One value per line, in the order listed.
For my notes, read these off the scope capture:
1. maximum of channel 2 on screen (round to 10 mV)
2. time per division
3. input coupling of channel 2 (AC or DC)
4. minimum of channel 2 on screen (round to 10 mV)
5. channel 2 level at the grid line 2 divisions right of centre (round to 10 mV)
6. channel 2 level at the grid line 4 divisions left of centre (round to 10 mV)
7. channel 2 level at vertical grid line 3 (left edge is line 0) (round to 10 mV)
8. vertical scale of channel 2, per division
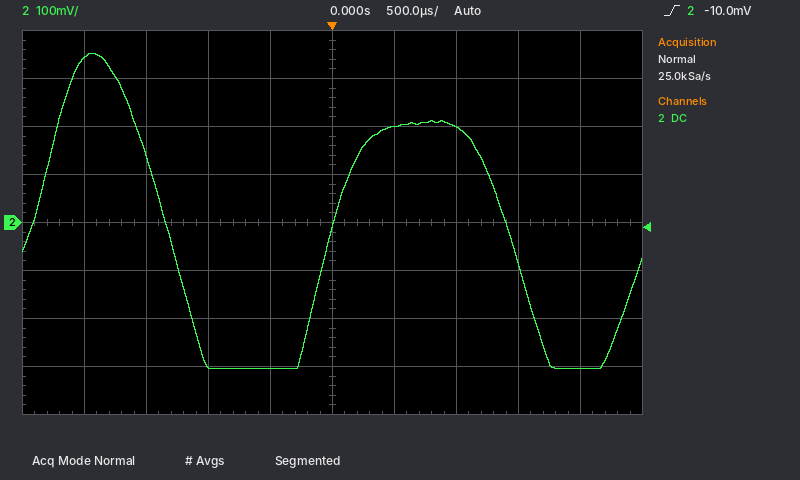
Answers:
350 mV
500 µs
DC
-300 mV
200 mV
340 mV
-300 mV
100 mV
